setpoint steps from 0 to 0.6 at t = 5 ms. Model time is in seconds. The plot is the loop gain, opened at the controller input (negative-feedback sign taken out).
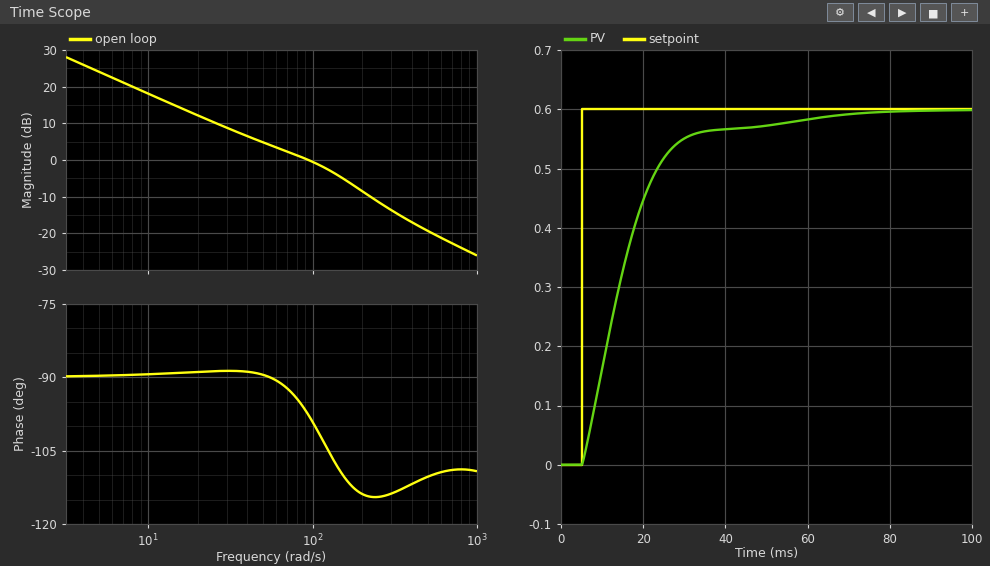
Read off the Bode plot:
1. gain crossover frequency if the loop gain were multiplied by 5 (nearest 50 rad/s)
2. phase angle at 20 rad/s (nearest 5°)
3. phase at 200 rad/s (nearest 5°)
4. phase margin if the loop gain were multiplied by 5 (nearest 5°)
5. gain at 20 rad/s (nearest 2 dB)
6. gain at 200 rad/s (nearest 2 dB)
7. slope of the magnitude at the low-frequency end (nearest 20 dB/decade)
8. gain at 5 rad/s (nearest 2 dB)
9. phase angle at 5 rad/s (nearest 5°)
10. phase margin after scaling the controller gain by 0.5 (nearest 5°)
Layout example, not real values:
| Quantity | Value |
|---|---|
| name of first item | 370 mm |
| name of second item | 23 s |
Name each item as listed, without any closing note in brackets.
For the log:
| Quantity | Value |
|---|---|
| gain crossover frequency if the loop gain were multiplied by 5 | 300 rad/s |
| phase angle at 20 rad/s | -90° |
| phase at 200 rad/s | -115° |
| phase margin if the loop gain were multiplied by 5 | 65° |
| gain at 20 rad/s | 12 dB |
| gain at 200 rad/s | -8 dB |
| slope of the magnitude at the low-frequency end | -20 dB/decade |
| gain at 5 rad/s | 24 dB |
| phase angle at 5 rad/s | -90° |
| phase margin after scaling the controller gain by 0.5 | 90° |
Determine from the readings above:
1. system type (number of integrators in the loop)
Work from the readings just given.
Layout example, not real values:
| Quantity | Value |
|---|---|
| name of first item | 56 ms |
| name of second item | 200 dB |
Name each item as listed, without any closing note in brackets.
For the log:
| Quantity | Value |
|---|---|
| system type | 1 |
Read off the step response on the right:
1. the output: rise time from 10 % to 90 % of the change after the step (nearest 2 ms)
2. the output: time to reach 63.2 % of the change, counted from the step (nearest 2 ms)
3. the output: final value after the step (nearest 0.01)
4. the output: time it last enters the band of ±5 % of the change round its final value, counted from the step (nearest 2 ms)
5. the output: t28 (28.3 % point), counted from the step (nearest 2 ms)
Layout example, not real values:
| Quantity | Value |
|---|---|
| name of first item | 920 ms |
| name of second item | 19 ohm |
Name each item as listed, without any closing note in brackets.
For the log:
| Quantity | Value |
|---|---|
| the output: rise time from 10 % to 90 % of the change after the step | 20 ms |
| the output: time to reach 63.2 % of the change, counted from the step | 12 ms |
| the output: final value after the step | 0.60 |
| the output: time it last enters the band of ±5 % of the change round its final value, counted from the step | 42 ms |
| the output: t28 (28.3 % point), counted from the step | 6 ms |
